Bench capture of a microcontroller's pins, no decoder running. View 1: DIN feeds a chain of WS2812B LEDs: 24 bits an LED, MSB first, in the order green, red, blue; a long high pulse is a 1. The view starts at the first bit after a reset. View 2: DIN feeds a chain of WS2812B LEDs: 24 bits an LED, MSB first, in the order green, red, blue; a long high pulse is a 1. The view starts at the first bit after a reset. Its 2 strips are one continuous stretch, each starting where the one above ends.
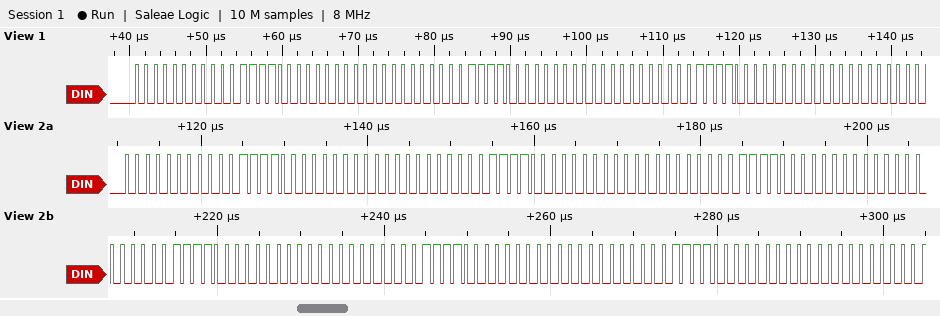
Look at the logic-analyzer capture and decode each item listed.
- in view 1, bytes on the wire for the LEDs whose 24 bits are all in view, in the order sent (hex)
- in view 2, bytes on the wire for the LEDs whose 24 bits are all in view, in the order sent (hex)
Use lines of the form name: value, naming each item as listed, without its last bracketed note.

in view 1, bytes on the wire for the LEDs whose 24 bits are all in view, in the order sent: 00 1E 00 00 1E 00 00 1E 00
in view 2, bytes on the wire for the LEDs whose 24 bits are all in view, in the order sent: 00 1E 00 00 1E 00 00 1E 00 00 1E 00 00 1E 00 00 1E 00
